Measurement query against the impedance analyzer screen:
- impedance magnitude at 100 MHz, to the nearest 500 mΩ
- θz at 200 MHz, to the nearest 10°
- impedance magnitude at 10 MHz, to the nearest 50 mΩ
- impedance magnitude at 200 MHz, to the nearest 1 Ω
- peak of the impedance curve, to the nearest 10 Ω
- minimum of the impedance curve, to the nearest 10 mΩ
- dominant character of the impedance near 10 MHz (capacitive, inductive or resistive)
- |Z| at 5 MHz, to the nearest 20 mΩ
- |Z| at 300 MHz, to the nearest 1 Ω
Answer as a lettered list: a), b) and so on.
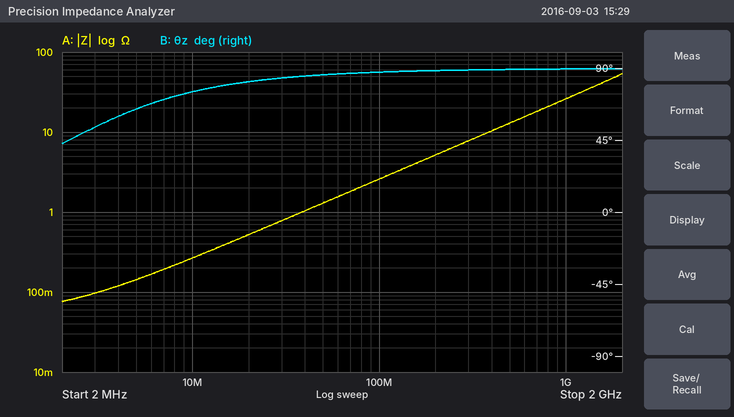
a) 2.5 Ω
b) 90°
c) 250 mΩ
d) 5 Ω
e) 50 Ω
f) 80 mΩ
g) inductive
h) 140 mΩ
i) 8 Ω
